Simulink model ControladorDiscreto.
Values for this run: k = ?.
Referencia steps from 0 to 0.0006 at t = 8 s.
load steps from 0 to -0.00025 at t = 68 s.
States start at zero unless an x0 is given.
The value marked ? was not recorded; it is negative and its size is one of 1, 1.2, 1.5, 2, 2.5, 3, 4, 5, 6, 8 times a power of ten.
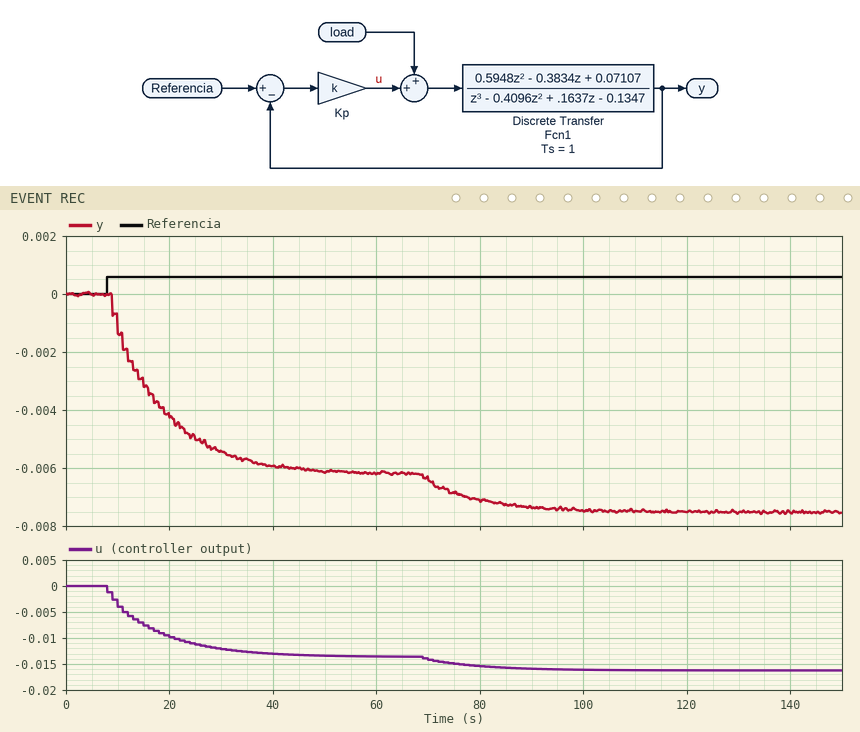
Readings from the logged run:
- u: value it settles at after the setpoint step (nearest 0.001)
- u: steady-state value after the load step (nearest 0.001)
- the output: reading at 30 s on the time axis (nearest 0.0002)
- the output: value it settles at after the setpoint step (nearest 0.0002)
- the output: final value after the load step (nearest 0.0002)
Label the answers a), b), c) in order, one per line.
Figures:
a) -0.014
b) -0.016
c) -0.0054
d) -0.0062
e) -0.0076
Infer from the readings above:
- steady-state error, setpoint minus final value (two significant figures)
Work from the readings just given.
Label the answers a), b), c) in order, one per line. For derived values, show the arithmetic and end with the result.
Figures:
a) 0.0006 - (-0.0062) = 0.0068
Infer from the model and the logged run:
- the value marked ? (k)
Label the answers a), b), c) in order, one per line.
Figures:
a) -2
